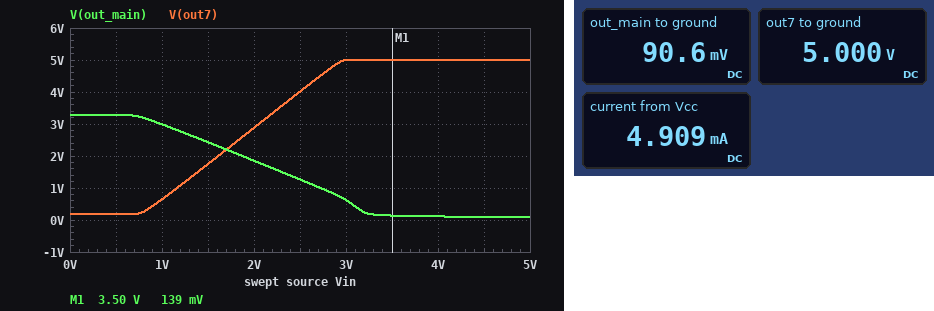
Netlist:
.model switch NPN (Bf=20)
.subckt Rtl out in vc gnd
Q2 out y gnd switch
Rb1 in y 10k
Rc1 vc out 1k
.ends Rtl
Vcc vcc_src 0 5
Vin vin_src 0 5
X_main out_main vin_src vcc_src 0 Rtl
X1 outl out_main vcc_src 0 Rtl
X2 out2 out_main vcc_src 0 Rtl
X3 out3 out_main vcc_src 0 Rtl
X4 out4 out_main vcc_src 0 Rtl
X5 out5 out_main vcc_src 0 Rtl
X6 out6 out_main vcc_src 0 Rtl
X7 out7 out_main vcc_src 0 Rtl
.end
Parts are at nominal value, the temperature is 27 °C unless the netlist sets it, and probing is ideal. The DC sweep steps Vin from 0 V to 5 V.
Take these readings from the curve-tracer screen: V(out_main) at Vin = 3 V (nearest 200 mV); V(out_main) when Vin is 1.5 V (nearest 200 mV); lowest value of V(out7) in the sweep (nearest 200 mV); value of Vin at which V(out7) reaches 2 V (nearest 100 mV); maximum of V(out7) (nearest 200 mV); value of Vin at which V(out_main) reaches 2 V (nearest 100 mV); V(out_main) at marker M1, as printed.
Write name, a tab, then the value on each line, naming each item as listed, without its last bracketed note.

V(out_main) at Vin = 3 V	600 mV
V(out_main) when Vin is 1.5 V	2.4 V
lowest value of V(out7) in the sweep	200 mV
value of Vin at which V(out7) reaches 2 V	1.6 V
maximum of V(out7)	5.0 V
value of Vin at which V(out_main) reaches 2 V	1.9 V
V(out_main) at marker M1, as printed	139 mV
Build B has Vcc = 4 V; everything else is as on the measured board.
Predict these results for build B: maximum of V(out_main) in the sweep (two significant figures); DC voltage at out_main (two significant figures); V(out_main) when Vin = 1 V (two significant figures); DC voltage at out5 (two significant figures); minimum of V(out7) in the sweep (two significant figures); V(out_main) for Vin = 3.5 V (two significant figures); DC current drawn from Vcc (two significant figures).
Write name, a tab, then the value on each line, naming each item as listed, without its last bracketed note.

maximum of V(out_main) in the sweep	2.7 V
DC voltage at out_main	79 mV
V(out_main) when Vin = 1 V	2.4 V
DC voltage at out5	4.0 V
minimum of V(out7) in the sweep	250 mV
V(out_main) for Vin = 3.5 V	110 mV
DC current drawn from Vcc	3.9 mA
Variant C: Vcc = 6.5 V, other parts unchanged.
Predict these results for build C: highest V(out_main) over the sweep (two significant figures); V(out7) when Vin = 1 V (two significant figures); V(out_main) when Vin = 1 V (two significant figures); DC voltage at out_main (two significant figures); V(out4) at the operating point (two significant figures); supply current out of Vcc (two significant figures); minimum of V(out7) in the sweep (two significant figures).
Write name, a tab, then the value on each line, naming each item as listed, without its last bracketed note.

highest V(out_main) over the sweep	4.2 V
V(out7) when Vin = 1 V	390 mV
V(out_main) when Vin = 1 V	3.9 V
DC voltage at out_main	110 mV
V(out4) at the operating point	6.5 V
supply current out of Vcc	6.4 mA
minimum of V(out7) in the sweep	160 mV
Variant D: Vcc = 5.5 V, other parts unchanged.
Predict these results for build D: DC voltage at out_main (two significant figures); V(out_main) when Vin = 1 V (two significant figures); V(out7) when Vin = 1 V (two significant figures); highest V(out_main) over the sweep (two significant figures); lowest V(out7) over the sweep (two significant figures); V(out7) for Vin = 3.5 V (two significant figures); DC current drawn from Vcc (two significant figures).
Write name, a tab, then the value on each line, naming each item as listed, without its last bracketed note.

DC voltage at out_main	97 mV
V(out_main) when Vin = 1 V	3.3 V
V(out7) when Vin = 1 V	560 mV
highest V(out_main) over the sweep	3.6 V
lowest V(out7) over the sweep	170 mV
V(out7) for Vin = 3.5 V	5.5 V
DC current drawn from Vcc	5.4 mA
